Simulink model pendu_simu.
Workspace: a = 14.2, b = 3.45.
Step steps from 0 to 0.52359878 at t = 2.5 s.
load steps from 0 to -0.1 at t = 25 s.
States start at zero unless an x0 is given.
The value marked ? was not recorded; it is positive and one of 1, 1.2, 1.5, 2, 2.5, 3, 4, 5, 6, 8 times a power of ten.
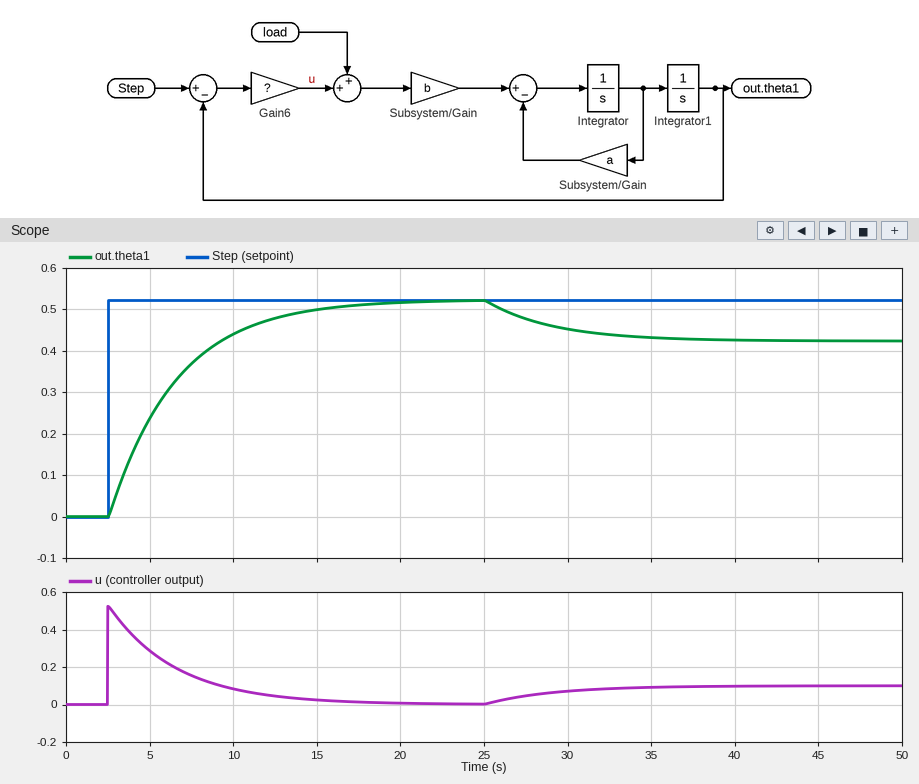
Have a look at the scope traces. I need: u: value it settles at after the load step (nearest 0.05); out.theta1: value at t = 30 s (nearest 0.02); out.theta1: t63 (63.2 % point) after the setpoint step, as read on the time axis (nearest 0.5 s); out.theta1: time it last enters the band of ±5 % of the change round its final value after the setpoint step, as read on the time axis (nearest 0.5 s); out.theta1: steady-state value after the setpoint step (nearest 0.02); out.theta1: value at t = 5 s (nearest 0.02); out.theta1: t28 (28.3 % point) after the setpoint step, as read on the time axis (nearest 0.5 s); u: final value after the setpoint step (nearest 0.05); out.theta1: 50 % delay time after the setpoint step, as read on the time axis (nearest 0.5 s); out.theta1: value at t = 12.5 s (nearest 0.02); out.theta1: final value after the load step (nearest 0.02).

0.10
0.46
6.5 s
14.5 s
0.52
0.24
4.0 s
0.00
5.5 s
0.48
0.42
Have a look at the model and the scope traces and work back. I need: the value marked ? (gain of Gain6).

1
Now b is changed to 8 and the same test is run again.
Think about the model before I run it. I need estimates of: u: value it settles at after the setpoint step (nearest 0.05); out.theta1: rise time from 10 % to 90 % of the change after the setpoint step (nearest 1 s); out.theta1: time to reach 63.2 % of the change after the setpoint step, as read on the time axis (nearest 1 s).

0.00
4 s
4 s
